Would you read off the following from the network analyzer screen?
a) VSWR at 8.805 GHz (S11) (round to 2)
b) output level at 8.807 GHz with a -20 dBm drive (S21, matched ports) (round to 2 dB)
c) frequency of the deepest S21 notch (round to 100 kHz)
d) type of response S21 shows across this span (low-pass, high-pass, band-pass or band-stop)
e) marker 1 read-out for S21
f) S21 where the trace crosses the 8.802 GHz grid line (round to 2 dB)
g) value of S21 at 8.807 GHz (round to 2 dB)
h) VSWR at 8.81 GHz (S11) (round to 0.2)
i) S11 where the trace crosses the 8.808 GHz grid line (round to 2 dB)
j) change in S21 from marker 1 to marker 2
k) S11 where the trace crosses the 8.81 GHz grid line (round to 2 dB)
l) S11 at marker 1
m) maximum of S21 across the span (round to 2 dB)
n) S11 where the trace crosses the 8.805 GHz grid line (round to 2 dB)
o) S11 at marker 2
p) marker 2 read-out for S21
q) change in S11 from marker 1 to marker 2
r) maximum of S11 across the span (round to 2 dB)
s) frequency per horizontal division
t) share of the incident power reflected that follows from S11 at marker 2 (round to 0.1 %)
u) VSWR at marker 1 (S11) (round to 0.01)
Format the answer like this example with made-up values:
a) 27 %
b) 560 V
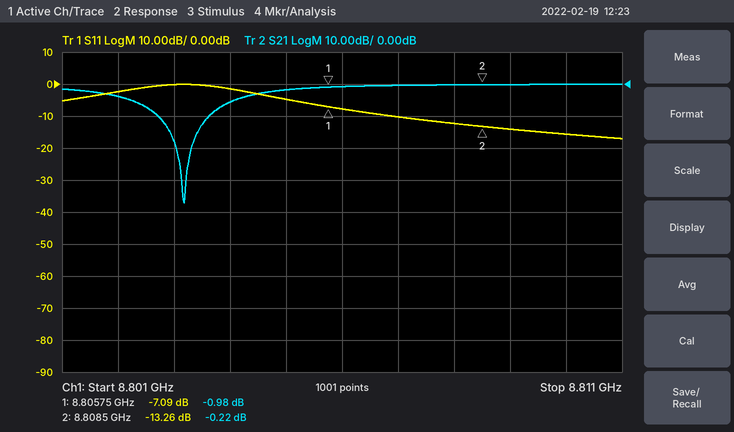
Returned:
a) 4
b) -20 dBm
c) 8.8032 GHz
d) band-stop
e) -0.98 dB
f) -4 dB
g) 0 dB
h) 1.4
i) -12 dB
j) 0.76 dB
k) -16 dB
l) -7.09 dB
m) 0 dB
n) -4 dB
o) -13.26 dB
p) -0.22 dB
q) -6.17 dB
r) 0 dB
s) 1 MHz
t) 4.7 %
u) 2.58
